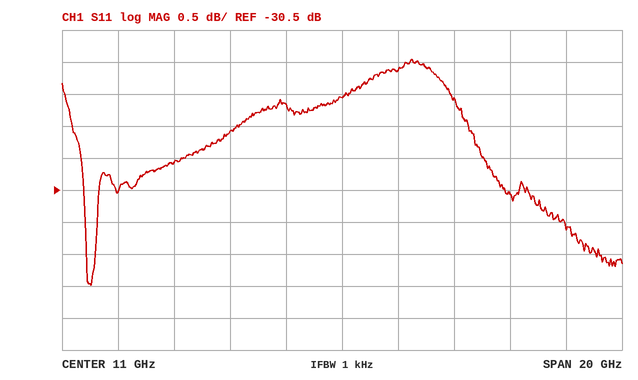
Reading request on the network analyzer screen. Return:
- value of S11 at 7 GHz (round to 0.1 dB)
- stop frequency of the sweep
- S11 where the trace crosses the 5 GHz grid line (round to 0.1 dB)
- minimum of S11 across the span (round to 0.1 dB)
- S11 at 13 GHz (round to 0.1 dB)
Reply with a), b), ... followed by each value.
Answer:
a) -29.6 dB
b) 21 GHz
c) -30.1 dB
d) -32.0 dB
e) -28.6 dB
